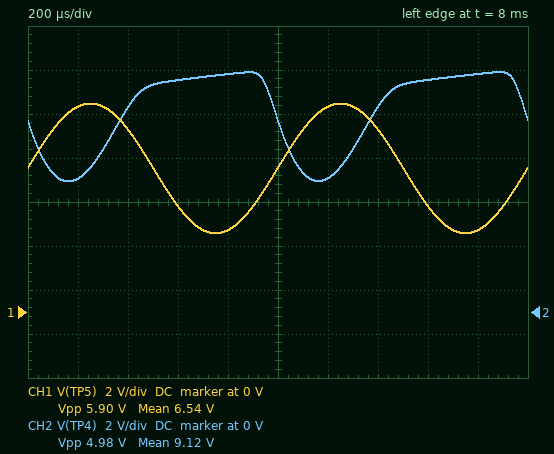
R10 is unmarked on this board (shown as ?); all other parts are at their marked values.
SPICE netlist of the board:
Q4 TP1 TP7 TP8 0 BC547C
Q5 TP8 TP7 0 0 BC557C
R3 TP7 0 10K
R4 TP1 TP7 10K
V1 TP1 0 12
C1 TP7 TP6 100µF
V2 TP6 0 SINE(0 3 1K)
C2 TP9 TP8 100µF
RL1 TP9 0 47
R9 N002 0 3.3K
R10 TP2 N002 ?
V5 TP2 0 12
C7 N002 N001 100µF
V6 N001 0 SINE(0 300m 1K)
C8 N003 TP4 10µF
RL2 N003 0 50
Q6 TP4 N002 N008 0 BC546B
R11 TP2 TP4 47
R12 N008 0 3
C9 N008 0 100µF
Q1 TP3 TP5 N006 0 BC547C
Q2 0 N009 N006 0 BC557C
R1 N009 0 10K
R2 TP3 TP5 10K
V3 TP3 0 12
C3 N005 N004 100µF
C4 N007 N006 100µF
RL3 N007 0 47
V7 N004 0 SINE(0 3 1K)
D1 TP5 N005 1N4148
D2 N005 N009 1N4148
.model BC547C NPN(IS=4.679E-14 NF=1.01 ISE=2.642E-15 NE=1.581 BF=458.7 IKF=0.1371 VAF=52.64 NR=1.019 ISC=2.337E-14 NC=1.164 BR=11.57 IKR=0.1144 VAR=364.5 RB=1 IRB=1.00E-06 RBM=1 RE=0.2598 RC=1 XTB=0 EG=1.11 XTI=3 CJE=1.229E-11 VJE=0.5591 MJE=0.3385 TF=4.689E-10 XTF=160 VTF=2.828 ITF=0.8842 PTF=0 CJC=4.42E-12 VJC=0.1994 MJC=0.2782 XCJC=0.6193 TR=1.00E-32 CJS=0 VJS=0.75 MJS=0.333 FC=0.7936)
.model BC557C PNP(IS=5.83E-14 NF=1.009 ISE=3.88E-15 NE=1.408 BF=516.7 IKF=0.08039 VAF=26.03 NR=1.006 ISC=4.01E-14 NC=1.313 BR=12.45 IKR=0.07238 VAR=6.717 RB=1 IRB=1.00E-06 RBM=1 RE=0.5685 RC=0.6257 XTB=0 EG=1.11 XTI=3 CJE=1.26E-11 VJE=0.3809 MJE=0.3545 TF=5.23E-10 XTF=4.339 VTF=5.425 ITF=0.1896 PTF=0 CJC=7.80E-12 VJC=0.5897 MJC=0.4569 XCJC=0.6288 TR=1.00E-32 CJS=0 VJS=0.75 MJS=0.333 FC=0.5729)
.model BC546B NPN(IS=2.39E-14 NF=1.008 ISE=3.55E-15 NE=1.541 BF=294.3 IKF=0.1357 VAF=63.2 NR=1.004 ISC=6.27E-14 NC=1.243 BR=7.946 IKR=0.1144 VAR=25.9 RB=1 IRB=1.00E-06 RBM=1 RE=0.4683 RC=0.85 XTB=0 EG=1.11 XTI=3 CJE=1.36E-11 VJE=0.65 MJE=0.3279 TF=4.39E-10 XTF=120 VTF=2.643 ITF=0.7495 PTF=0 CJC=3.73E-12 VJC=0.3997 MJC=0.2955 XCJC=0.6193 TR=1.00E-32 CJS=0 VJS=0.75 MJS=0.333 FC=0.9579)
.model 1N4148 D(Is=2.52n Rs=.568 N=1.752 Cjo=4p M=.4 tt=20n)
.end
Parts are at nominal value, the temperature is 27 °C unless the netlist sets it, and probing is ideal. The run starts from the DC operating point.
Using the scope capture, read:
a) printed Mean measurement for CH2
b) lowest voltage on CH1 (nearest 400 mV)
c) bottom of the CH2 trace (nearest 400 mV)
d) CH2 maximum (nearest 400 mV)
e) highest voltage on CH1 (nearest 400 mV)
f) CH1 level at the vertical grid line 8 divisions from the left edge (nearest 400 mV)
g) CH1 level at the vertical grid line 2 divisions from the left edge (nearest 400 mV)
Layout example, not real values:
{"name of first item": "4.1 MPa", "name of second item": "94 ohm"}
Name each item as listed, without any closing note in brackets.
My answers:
{"printed Mean measurement for CH2": "9.12 V", "lowest voltage on CH1": "3.6 V", "bottom of the CH2 trace": "6.0 V", "CH2 maximum": "10.8 V", "highest voltage on CH1": "9.6 V", "CH1 level at the vertical grid line 8 divisions from the left edge": "4.8 V", "CH1 level at the vertical grid line 2 divisions from the left edge": "8.4 V"}
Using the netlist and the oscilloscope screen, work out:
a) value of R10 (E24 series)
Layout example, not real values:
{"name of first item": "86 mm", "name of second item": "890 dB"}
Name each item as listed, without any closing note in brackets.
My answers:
{"value of R10": "24 kΩ"}
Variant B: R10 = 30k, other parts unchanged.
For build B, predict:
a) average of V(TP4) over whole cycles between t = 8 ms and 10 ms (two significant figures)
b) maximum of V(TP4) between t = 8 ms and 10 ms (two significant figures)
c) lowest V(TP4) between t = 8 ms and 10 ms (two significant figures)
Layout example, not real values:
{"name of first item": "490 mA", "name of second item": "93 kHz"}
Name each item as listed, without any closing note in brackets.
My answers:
{"average of V(TP4) over whole cycles between t = 8 ms and 10 ms": "9.6 V", "maximum of V(TP4) between t = 8 ms and 10 ms": "11 V", "lowest V(TP4) between t = 8 ms and 10 ms": "6.7 V"}
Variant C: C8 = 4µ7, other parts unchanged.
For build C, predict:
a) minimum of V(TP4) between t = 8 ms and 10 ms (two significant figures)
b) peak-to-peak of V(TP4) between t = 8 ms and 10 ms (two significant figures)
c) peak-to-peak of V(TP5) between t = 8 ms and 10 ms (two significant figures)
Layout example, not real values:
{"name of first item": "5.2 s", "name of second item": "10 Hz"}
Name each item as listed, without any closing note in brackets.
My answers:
{"minimum of V(TP4) between t = 8 ms and 10 ms": "5.7 V", "peak-to-peak of V(TP4) between t = 8 ms and 10 ms": "5.5 V", "peak-to-peak of V(TP5) between t = 8 ms and 10 ms": "5.9 V"}
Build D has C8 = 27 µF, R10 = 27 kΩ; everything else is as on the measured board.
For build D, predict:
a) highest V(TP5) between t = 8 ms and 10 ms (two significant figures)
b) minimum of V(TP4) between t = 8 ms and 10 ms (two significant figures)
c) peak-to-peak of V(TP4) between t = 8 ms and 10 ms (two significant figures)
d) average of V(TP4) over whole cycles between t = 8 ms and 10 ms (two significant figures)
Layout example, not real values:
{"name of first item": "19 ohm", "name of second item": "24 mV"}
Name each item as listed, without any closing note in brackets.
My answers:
{"highest V(TP5) between t = 8 ms and 10 ms": "9.5 V", "minimum of V(TP4) between t = 8 ms and 10 ms": "6.4 V", "peak-to-peak of V(TP4) between t = 8 ms and 10 ms": "4.5 V", "average of V(TP4) over whole cycles between t = 8 ms and 10 ms": "9.4 V"}
